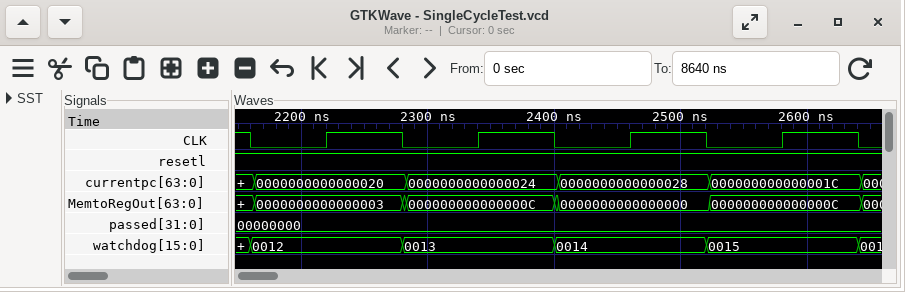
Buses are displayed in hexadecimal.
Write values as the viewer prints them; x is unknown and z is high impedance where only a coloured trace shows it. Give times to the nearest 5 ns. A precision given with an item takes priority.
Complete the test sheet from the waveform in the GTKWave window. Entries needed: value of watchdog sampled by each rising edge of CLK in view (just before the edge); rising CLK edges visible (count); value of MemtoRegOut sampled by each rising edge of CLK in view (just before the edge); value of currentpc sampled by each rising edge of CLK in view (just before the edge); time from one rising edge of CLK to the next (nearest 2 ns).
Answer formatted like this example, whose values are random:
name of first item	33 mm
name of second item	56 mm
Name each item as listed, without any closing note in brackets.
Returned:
value of watchdog sampled by each rising edge of CLK in view	0012, 0013, 0014, 0015
rising CLK edges visible	4
value of MemtoRegOut sampled by each rising edge of CLK in view	0000000000000003, 000000000000000C, 0000000000000000, 000000000000000C
value of currentpc sampled by each rising edge of CLK in view	0000000000000020, 0000000000000024, 0000000000000028, 000000000000001C
time from one rising edge of CLK to the next	120 ns
